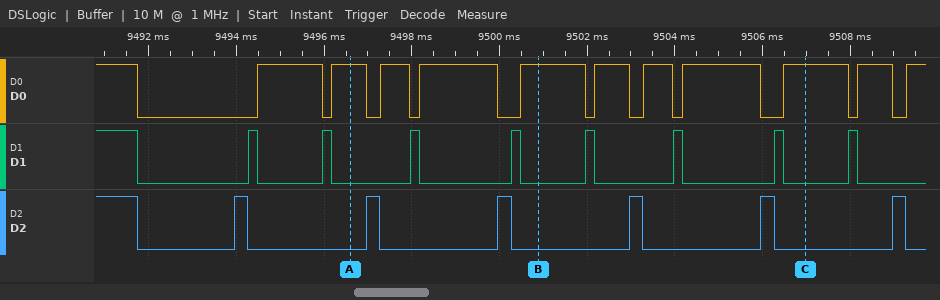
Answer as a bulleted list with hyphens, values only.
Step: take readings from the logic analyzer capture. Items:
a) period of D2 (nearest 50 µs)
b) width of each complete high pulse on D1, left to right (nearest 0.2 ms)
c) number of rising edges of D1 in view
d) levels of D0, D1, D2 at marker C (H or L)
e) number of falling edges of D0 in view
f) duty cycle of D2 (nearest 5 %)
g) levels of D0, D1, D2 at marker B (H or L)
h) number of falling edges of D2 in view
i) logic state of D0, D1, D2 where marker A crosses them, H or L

- 3000 µs
- 0.2 ms, 0.2 ms, 0.2 ms, 0.2 ms, 0.2 ms, 0.2 ms, 0.2 ms, 0.2 ms
- 8
- D0=H, D1=L, D2=L
- 11
- 10 %
- D0=H, D1=L, D2=L
- 7
- D0=H, D1=L, D2=L
